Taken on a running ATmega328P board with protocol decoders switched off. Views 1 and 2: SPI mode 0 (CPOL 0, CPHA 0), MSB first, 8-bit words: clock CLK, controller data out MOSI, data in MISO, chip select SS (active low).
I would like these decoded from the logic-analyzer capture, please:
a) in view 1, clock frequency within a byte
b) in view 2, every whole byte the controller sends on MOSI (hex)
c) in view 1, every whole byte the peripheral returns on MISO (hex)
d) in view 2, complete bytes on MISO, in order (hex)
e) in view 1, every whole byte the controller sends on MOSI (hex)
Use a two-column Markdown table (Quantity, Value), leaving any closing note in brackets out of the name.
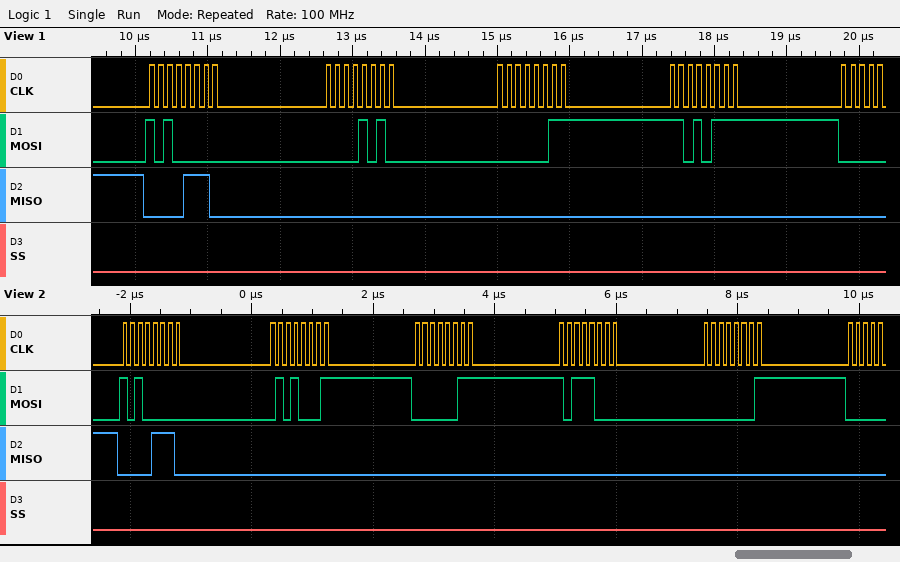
| Quantity | Value |
|---|---|
| in view 1, clock frequency within a byte | 8 MHz |
| in view 2, every whole byte the controller sends on MOSI | A0 51 03 B8 01 |
| in view 1, every whole byte the peripheral returns on MISO | 0E 00 00 00 |
| in view 2, complete bytes on MISO, in order | 0E 00 00 00 00 |
| in view 1, every whole byte the controller sends on MOSI | A0 0A 03 D7 |
